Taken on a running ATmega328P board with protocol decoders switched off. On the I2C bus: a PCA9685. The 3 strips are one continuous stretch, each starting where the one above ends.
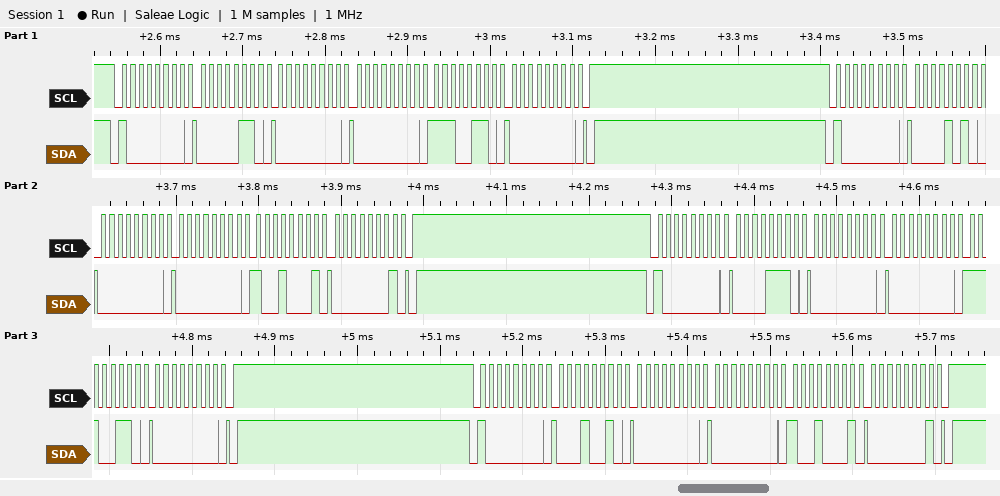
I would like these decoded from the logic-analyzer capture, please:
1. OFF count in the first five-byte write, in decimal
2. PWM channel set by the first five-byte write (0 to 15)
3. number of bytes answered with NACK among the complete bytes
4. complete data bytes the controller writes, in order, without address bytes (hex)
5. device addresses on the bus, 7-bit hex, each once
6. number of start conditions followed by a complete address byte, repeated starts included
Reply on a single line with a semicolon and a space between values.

230; 0; 0; 06 00 00 E6 00 0A 00 00 91 01 0E 00 00 E6 00 12 00 00 91 01; 0x40; 4
